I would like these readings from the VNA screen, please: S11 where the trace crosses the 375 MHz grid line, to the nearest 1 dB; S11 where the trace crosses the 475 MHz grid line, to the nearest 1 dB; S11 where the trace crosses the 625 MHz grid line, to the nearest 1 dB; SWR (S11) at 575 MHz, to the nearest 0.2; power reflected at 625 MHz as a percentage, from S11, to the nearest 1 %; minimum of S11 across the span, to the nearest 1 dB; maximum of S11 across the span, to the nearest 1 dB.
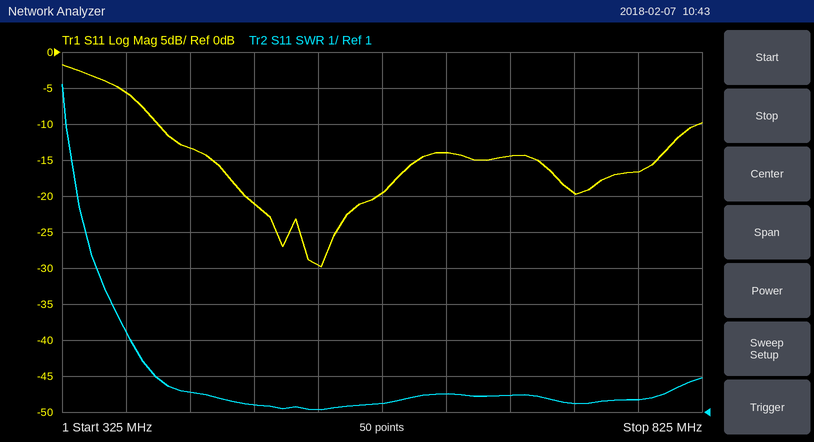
-6 dB
-21 dB
-14 dB
1.2
4 %
-30 dB
-2 dB
